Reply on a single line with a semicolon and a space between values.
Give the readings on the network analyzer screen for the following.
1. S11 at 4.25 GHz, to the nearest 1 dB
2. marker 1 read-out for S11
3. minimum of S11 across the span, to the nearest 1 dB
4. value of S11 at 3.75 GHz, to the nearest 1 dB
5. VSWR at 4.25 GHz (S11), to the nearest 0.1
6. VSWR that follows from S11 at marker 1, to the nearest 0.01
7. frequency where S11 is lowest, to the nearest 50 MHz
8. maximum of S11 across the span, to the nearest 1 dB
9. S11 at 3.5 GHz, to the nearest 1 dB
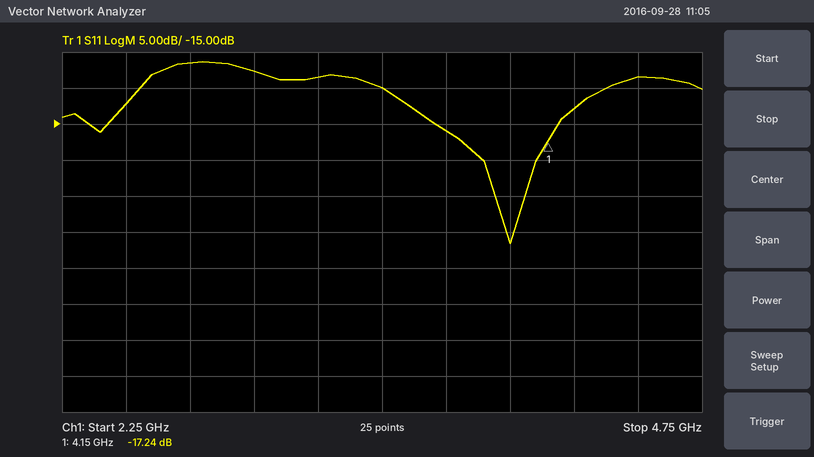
-13 dB; -17.24 dB; -32 dB; -16 dB; 1.6; 1.32; 4.00 GHz; -6 dB; -10 dB
